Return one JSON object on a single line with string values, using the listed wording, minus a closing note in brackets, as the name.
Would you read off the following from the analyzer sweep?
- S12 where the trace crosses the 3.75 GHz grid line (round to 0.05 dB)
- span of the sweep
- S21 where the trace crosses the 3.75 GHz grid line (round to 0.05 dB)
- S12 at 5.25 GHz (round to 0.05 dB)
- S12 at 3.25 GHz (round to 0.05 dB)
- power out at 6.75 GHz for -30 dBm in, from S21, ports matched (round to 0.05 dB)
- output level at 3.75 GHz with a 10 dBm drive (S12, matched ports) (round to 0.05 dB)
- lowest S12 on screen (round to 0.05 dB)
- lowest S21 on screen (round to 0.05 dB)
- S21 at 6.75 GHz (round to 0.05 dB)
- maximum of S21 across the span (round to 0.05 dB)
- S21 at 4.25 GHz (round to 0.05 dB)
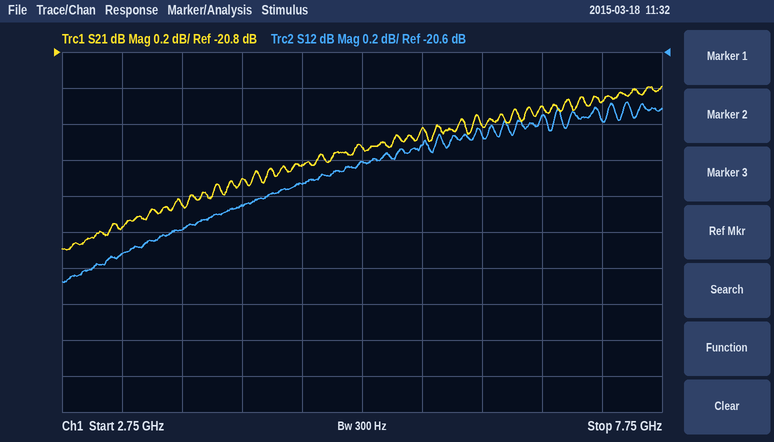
{"S12 where the trace crosses the 3.75 GHz grid line": "-21.60 dB", "span of the sweep": "5 GHz", "S21 where the trace crosses the 3.75 GHz grid line": "-21.65 dB", "S12 at 5.25 GHz": "-21.20 dB", "S12 at 3.25 GHz": "-21.70 dB", "power out at 6.75 GHz for -30 dBm in, from S21, ports matched": "-51.10 dBm", "output level at 3.75 GHz with a 10 dBm drive (S12, matched ports)": "-11.60 dBm", "lowest S12 on screen": "-21.90 dB", "lowest S21 on screen": "-21.90 dB", "S21 at 6.75 GHz": "-21.10 dB", "maximum of S21 across the span": "-21.00 dB", "S21 at 4.25 GHz": "-21.50 dB"}
